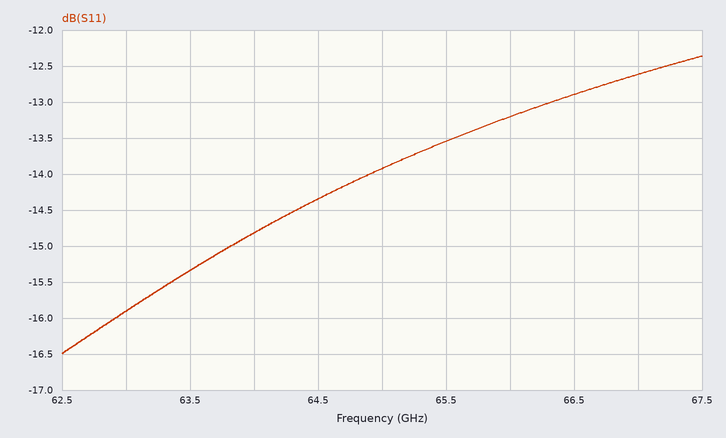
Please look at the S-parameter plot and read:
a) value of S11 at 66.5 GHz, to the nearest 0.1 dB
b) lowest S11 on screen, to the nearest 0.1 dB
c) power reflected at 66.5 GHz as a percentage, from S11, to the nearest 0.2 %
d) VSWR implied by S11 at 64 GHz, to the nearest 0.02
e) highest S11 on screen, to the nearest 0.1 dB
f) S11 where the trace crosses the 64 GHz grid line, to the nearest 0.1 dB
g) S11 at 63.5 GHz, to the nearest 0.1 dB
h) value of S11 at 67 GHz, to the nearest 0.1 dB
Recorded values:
-12.9 dB
-16.5 dB
5.2 %
1.44
-12.4 dB
-14.8 dB
-15.3 dB
-12.6 dB
